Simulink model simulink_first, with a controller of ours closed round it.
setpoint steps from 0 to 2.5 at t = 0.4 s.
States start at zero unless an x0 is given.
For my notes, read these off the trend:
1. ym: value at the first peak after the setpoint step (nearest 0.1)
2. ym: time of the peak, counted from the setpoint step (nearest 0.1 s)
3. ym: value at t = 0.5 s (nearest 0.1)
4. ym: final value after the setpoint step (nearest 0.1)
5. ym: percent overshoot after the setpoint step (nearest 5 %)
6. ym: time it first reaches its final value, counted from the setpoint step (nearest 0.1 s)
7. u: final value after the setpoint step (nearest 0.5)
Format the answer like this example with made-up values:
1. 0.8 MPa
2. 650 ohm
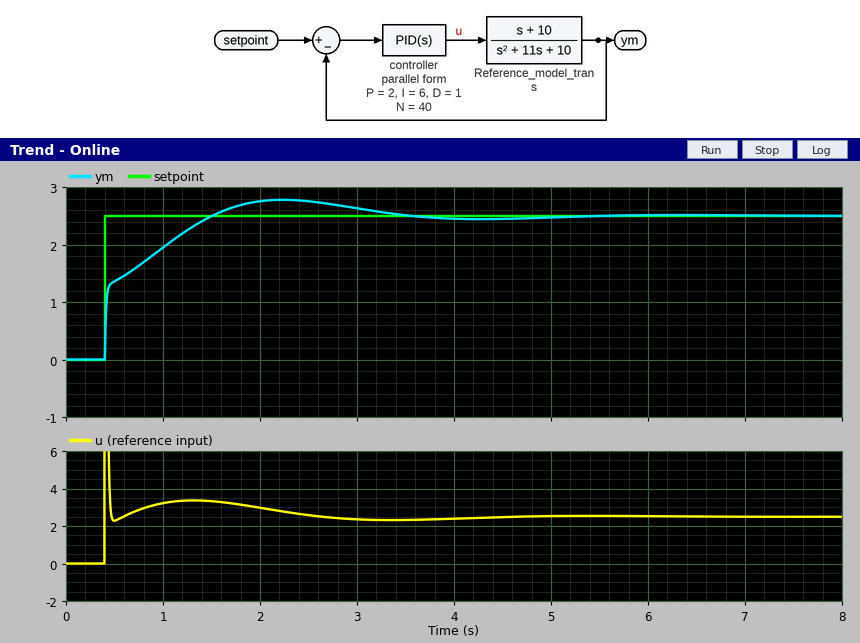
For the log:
1. 2.8
2. 1.8 s
3. 1.4
4. 2.5
5. 10 %
6. 1.1 s
7. 2.5
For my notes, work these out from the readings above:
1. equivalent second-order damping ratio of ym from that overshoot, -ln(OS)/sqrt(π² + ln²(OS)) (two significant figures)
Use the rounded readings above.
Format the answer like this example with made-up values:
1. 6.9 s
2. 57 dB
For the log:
1. 0.59
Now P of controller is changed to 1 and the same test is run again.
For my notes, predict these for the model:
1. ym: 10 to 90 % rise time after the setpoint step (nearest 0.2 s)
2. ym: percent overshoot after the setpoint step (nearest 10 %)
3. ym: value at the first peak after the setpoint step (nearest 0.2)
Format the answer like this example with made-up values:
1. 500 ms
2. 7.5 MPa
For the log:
1. 1.0 s
2. 20 %
3. 3.0
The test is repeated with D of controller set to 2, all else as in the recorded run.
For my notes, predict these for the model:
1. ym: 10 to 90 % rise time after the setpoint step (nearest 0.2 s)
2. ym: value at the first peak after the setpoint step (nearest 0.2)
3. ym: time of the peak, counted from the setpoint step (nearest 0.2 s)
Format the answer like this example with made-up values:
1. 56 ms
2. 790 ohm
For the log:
1. 1.0 s
2. 2.8
3. 2.4 s
